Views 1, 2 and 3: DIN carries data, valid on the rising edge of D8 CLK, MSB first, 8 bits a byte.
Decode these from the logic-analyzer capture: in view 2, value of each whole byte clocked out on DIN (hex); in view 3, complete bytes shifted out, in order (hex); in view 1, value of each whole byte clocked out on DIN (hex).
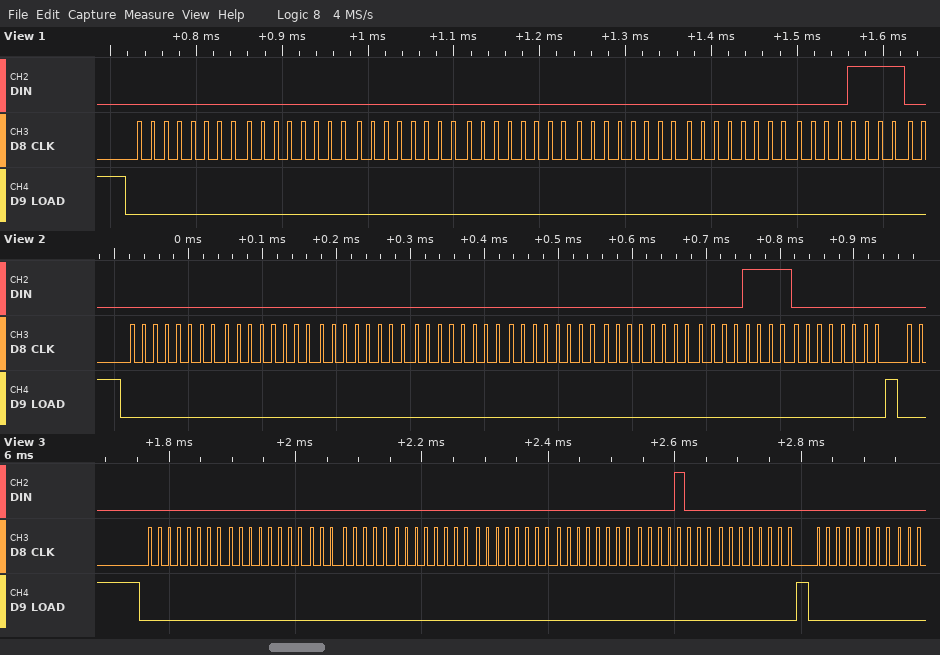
0x00 0x00 0x00 0x00 0x00 0x00 0x0F 0x00
00 00 00 00 00 00 08 00 00
00 00 00 00 00 00 0F
